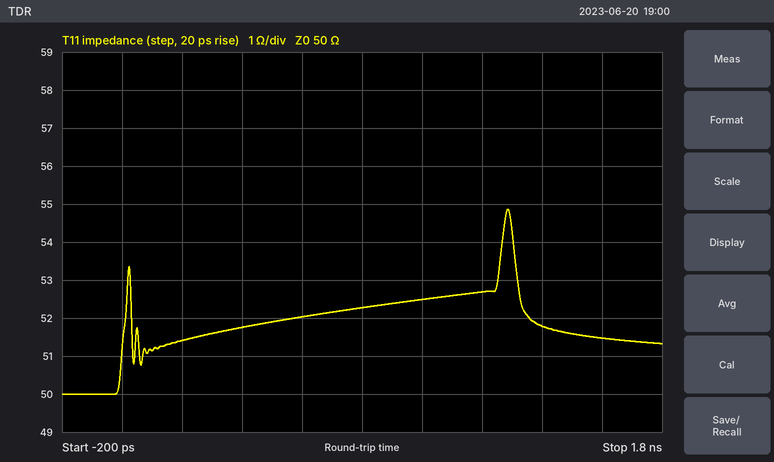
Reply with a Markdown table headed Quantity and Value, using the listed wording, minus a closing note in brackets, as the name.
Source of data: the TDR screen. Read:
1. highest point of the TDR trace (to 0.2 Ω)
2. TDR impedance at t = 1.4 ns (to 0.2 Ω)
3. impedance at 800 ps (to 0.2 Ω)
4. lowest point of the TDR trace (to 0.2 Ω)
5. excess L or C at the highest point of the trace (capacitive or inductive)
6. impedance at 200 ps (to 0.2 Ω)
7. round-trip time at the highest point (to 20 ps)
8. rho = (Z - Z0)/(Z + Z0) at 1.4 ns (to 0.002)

| Quantity | Value |
|---|---|
| highest point of the TDR trace | 54.8 Ω |
| TDR impedance at t = 1.4 ns | 51.8 Ω |
| impedance at 800 ps | 52.2 Ω |
| lowest point of the TDR trace | 50.0 Ω |
| excess L or C at the highest point of the trace | inductive |
| impedance at 200 ps | 51.4 Ω |
| round-trip time at the highest point | 1.28 ns |
| rho = (Z - Z0)/(Z + Z0) at 1.4 ns | +0.018 |
